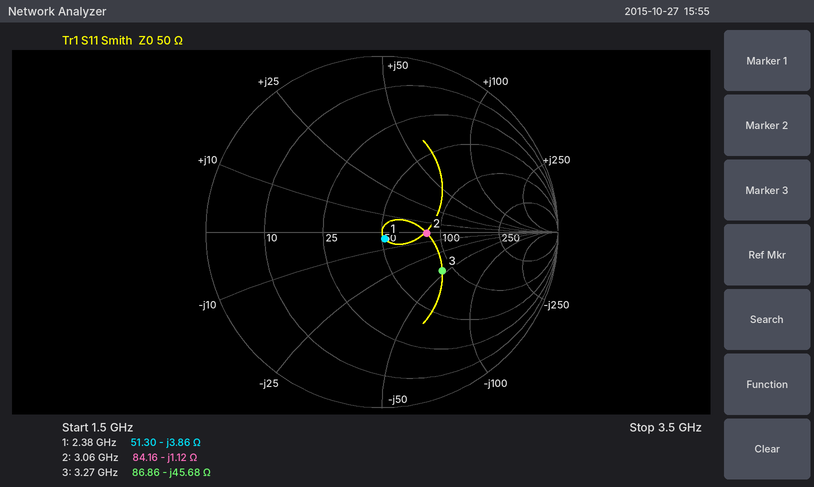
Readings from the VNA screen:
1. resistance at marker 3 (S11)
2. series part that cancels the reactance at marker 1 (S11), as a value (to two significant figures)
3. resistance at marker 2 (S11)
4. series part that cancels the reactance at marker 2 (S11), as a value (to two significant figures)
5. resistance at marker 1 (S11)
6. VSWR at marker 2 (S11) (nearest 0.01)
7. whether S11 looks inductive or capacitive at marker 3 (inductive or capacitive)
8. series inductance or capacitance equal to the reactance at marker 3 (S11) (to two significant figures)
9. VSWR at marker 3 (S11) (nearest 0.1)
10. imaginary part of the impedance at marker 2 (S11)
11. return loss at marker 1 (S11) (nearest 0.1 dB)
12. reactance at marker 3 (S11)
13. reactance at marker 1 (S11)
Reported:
86.86 Ω
260 pH
84.16 Ω
58 pH
51.30 Ω
1.68
capacitive
1.1 pF
2.4
-1.12 Ω
27.9 dB
-45.68 Ω
-3.86 Ω
